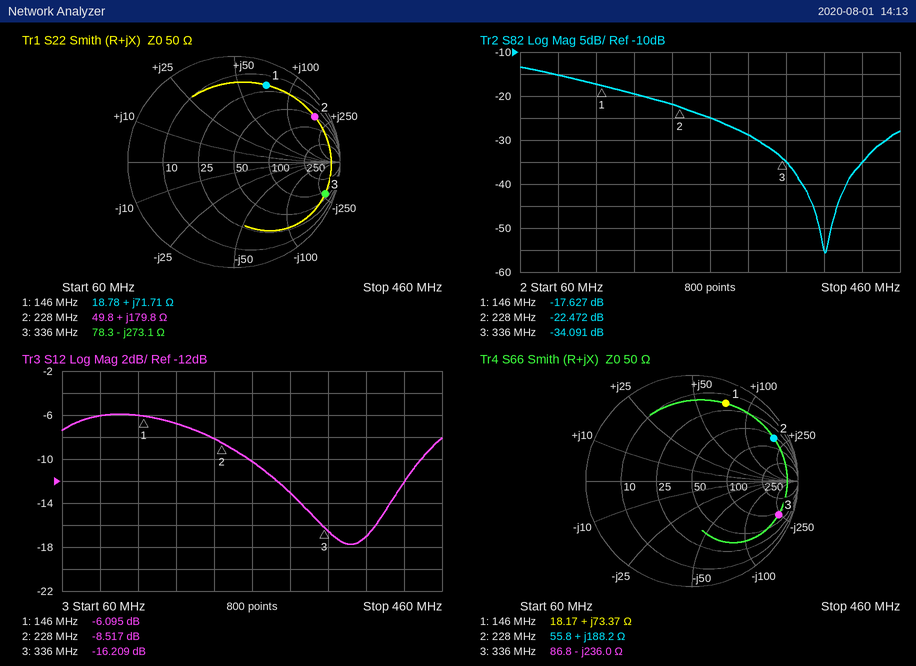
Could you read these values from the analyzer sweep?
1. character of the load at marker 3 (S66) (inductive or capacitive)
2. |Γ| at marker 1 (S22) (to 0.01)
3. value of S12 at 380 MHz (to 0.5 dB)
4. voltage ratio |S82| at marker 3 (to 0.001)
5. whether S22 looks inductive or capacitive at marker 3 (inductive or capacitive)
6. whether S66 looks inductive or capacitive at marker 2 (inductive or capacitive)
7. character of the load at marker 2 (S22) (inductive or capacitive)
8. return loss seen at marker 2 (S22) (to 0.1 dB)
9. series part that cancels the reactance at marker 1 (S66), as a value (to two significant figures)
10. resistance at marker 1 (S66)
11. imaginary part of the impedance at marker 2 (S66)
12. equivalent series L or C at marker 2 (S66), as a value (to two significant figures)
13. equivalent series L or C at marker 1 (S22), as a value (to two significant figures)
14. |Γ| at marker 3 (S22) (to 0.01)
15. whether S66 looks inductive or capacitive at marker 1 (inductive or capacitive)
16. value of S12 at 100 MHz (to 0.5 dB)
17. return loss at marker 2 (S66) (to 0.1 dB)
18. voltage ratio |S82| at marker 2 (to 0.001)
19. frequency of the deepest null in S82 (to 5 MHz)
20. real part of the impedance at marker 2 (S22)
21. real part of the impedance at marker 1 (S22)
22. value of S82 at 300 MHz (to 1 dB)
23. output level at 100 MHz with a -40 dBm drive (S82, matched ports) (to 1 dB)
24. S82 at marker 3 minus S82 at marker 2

capacitive
0.79
-17.0 dB
0.020
capacitive
inductive
inductive
1.2 dB
15 pF
18.17 Ω
+188.2 Ω
130 nH
78 nH
0.91
inductive
-6.0 dB
1.2 dB
0.075
380 MHz
49.8 Ω
18.78 Ω
-29 dB
-55 dBm
-11.619 dB
